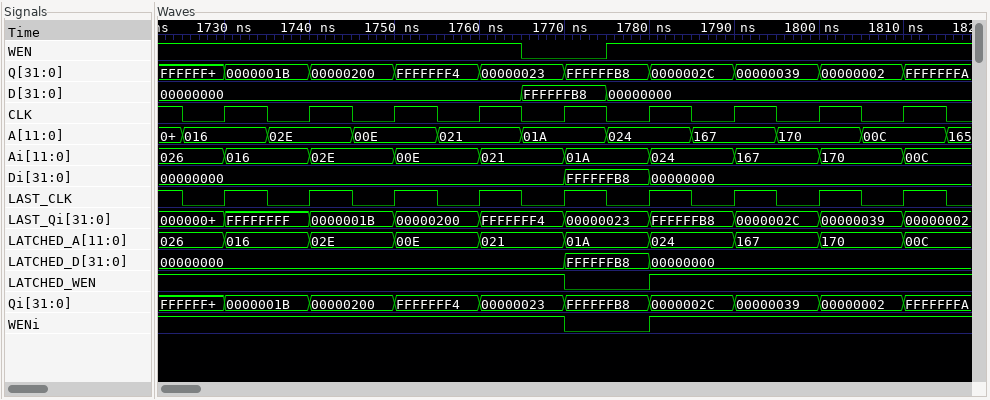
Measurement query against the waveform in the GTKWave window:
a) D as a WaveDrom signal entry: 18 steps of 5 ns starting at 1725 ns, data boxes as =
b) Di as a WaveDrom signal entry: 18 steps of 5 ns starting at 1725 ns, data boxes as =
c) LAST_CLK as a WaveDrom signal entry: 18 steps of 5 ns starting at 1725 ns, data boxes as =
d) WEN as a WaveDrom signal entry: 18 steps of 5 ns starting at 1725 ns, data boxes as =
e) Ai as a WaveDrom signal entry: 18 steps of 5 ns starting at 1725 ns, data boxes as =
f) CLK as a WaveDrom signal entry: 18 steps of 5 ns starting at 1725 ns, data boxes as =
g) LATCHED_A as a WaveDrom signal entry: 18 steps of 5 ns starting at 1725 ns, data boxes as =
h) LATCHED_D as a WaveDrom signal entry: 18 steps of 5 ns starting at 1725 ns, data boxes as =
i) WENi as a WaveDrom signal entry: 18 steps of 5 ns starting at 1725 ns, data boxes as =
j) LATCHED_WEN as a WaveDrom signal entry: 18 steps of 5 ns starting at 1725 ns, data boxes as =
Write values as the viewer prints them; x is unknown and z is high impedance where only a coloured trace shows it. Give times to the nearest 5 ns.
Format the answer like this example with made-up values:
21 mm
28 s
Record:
{name: 'D', wave: '=.......=.=.......', data: '00000000 FFFFFFB8 00000000'}
{name: 'Di', wave: '=........=.=......', data: '00000000 FFFFFFB8 00000000'}
{name: 'LAST_CLK', wave: '010101010101010101'}
{name: 'WEN', wave: '1.......0.1.......'}
{name: 'Ai', wave: '==.=.=.=.=.=.=.=.=', data: '026 016 02E 00E 021 01A 024 167 170 00C'}
{name: 'CLK', wave: '010101010101010101'}
{name: 'LATCHED_A', wave: '==.=.=.=.=.=.=.=.=', data: '026 016 02E 00E 021 01A 024 167 170 00C'}
{name: 'LATCHED_D', wave: '=........=.=......', data: '00000000 FFFFFFB8 00000000'}
{name: 'WENi', wave: '1........0.1......'}
{name: 'LATCHED_WEN', wave: '1........0.1......'}
